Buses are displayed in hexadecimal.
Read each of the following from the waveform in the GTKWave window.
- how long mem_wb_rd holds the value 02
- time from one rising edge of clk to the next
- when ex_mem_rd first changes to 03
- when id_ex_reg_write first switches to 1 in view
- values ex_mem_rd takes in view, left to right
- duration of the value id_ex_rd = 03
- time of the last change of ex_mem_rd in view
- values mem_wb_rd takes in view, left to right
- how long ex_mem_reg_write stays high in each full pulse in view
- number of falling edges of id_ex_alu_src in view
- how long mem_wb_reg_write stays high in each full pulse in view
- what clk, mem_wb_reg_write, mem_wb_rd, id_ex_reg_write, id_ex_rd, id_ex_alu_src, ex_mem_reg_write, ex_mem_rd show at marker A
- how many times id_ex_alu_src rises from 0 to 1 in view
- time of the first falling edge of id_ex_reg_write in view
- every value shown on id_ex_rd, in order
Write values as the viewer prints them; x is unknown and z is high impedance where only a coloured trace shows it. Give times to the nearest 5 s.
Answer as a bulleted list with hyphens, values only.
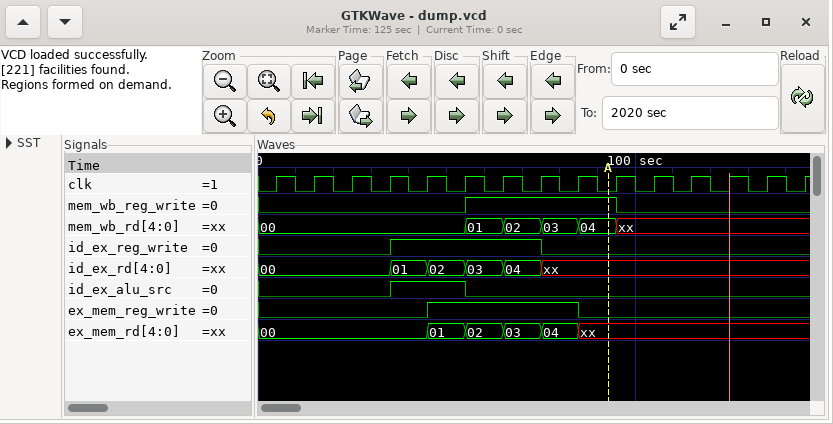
- 10 s
- 10 s
- 65 s
- 35 s
- 00, 01, 02, 03, 04, xx
- 10 s
- 85 s
- 00, 01, 02, 03, 04, xx
- 40 s
- 1
- 40 s
- clk=0, mem_wb_reg_write=1, mem_wb_rd=04, id_ex_reg_write=0, id_ex_rd=xx, id_ex_alu_src=0, ex_mem_reg_write=0, ex_mem_rd=xx
- 1
- 75 s
- 00, 01, 02, 03, 04, xx
